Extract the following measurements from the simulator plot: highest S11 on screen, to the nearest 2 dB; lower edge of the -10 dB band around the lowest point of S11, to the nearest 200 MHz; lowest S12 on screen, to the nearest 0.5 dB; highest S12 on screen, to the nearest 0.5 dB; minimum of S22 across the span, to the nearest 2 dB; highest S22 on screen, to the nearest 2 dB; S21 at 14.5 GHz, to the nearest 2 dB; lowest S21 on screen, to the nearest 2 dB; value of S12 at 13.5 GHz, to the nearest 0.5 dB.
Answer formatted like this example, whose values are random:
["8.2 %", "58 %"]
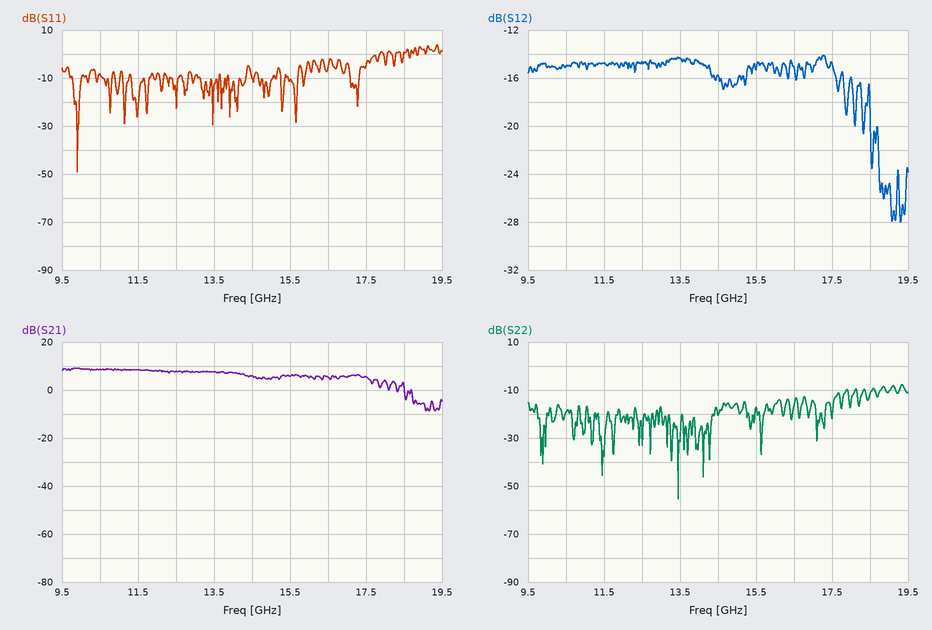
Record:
["4 dB", "9.8 GHz", "-28.0 dB", "-14.0 dB", "-56 dB", "-8 dB", "6 dB", "-8 dB", "-14.5 dB"]
